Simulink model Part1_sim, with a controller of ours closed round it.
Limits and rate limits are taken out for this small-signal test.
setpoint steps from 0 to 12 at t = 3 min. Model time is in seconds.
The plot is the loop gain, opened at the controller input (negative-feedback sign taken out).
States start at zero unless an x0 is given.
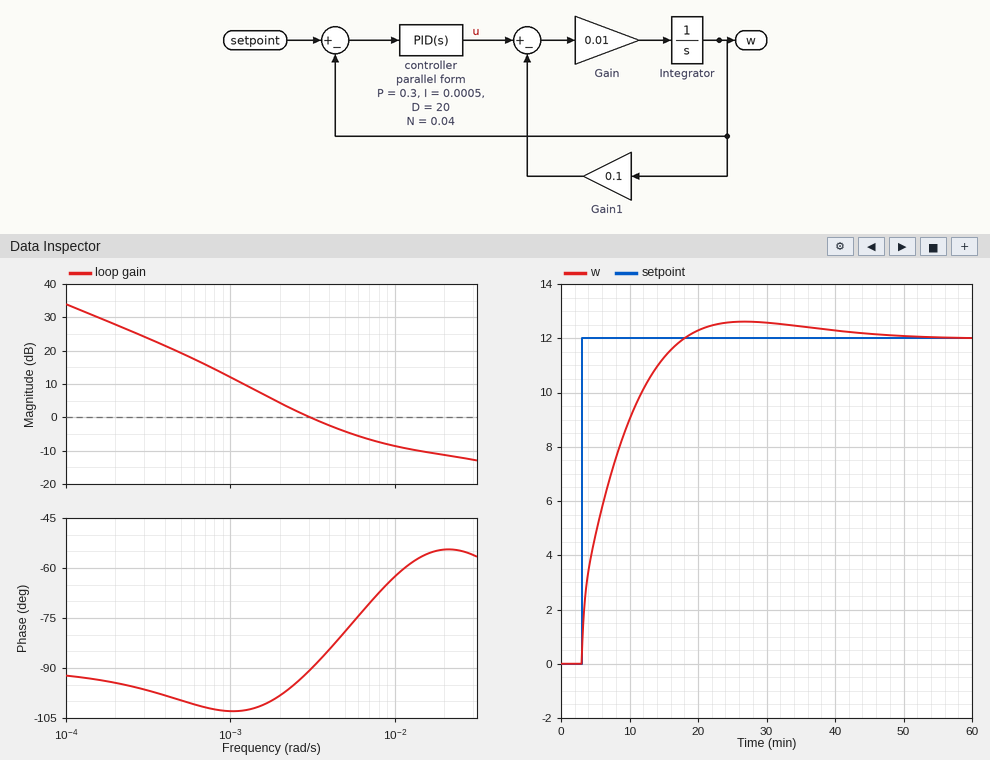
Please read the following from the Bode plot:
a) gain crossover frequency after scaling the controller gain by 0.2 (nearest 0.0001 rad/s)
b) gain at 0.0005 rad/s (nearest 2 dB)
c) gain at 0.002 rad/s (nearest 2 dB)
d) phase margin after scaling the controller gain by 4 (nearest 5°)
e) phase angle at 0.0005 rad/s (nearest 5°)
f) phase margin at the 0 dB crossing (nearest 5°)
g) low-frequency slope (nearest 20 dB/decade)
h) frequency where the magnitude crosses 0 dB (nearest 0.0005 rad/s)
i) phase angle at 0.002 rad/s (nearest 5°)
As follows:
0.0008 rad/s
20 dB
4 dB
125°
-100°
90°
-20 dB/decade
0.0030 rad/s
-100°
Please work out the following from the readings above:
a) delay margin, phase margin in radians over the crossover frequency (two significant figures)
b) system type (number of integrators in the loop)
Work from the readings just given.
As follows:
520 s
1
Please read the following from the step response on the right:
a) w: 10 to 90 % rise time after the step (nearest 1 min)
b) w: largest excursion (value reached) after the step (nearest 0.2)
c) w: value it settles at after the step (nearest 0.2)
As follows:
10 min
12.6
12.0
